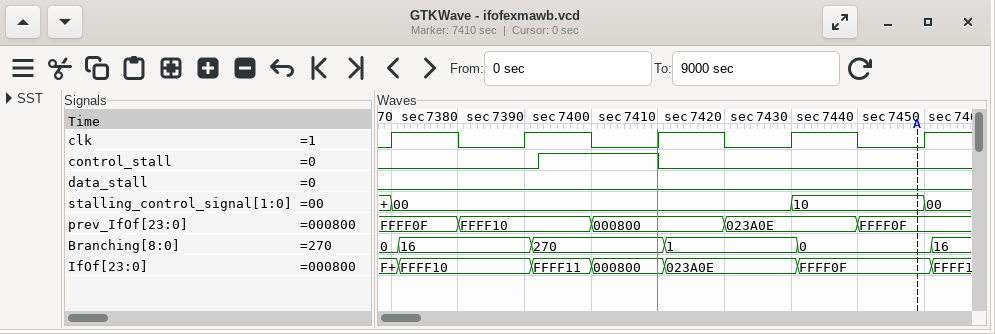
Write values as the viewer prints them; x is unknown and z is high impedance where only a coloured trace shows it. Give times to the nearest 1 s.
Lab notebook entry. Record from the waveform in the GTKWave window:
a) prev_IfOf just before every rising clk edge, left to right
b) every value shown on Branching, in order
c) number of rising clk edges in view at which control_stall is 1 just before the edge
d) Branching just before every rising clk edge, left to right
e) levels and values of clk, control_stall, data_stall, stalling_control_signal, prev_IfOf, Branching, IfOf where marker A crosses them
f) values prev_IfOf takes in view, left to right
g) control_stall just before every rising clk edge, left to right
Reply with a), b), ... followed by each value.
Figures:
a) FFFF0F, FFFF10, 000800, 023A0E, FFFF0F
b) 0, 16, 270, 1, 0, 16
c) 1
d) 0, 16, 270, 1, 0
e) clk=0, control_stall=0, data_stall=0, stalling_control_signal=10, prev_IfOf=FFFF0F, Branching=0, IfOf=FFFF0F
f) FFFF0F, FFFF10, 000800, 023A0E, FFFF0F
g) 0 0 1 0 0
